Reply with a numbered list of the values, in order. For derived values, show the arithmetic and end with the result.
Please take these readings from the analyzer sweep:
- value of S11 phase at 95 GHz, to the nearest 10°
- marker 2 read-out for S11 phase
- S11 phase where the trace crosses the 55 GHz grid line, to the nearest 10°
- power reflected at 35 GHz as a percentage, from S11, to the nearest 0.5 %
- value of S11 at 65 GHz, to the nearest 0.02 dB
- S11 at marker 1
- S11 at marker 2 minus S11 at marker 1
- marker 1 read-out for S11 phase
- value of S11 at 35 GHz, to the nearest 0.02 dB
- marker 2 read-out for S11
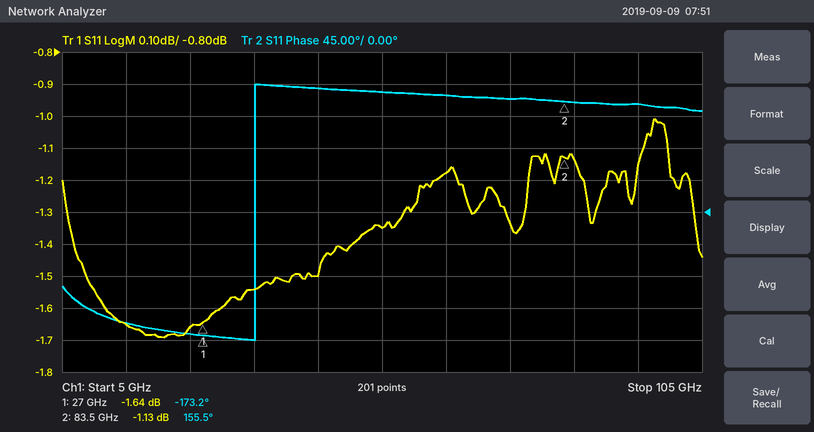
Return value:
1. 150°
2. 155.5°
3. 170°
4. 10^(-1.54/10) ≈ 70.1 %, so 70.0 % to the nearest 0.5 %
5. -1.18 dB
6. -1.64 dB
7. -1.13 − (-1.64) = 0.51 dB
8. -173.2°
9. -1.54 dB
10. -1.13 dB
